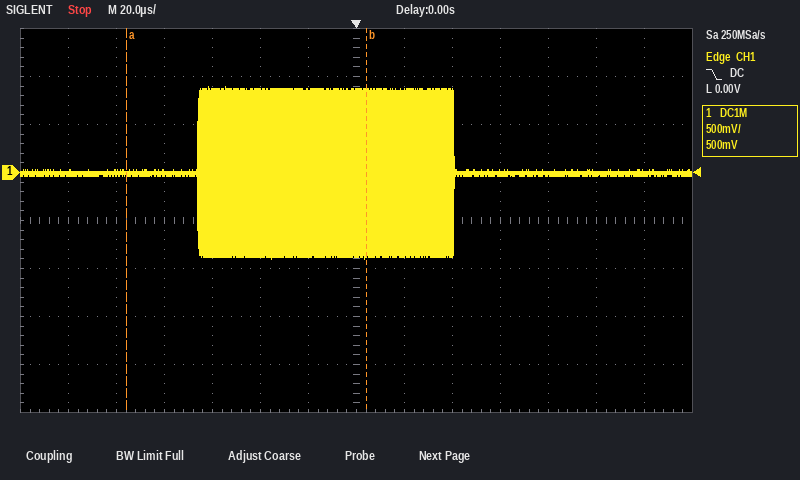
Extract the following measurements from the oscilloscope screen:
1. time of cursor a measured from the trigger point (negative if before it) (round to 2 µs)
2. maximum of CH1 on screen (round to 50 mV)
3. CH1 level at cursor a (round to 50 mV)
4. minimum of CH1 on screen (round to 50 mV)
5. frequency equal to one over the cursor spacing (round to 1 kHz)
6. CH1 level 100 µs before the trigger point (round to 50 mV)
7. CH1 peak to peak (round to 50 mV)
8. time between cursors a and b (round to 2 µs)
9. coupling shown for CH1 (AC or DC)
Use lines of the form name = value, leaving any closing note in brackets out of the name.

time of cursor a measured from the trigger point (negative if before it) = -96 µs
maximum of CH1 on screen = 900 mV
CH1 level at cursor a = 0 mV
minimum of CH1 on screen = -900 mV
frequency equal to one over the cursor spacing = 10 kHz
CH1 level 100 µs before the trigger point = 0 mV
CH1 peak to peak = 1.80 V
time between cursors a and b = 100 µs
coupling shown for CH1 = DC
